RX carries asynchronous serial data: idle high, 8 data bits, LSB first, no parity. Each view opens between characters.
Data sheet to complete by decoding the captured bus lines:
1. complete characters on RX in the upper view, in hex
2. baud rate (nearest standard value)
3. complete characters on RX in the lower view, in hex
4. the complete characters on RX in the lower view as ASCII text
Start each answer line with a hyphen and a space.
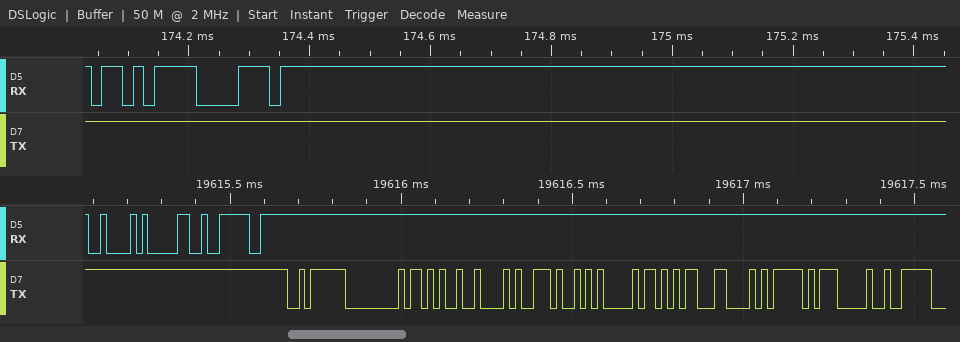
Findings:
- EB, B8
- 57600 baud
- 42, 30, 3E
- "B0>"
